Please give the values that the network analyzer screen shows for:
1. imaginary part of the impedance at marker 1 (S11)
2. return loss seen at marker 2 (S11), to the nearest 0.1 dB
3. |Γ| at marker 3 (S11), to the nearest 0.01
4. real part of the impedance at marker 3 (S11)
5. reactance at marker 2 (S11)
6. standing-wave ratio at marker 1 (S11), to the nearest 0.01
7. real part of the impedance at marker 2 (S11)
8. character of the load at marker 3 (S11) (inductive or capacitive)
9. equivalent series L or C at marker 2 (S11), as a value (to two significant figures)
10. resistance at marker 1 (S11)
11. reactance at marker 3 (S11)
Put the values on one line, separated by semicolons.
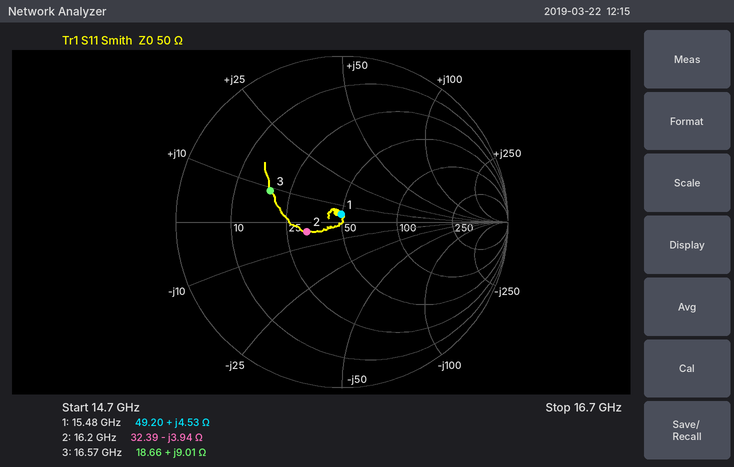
+4.53 Ω; 13.2 dB; 0.47; 18.66 Ω; -3.94 Ω; 1.10; 32.39 Ω; inductive; 2.5 pF; 49.20 Ω; +9.01 Ω
